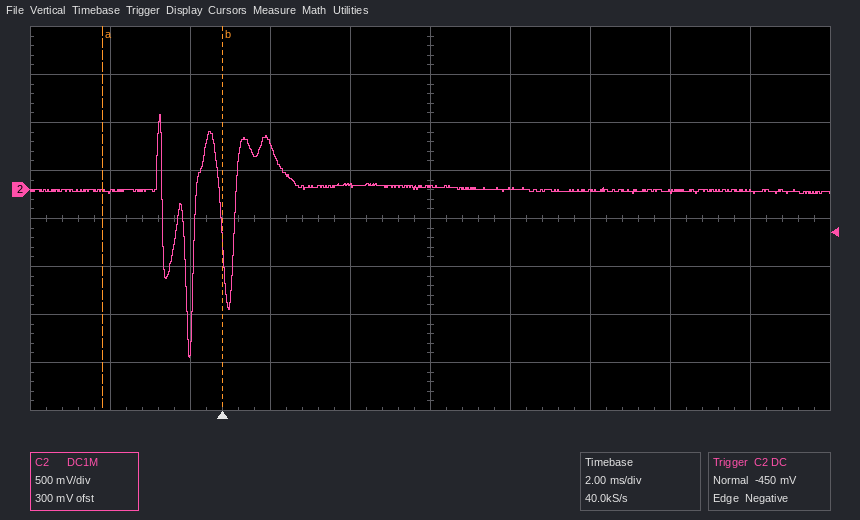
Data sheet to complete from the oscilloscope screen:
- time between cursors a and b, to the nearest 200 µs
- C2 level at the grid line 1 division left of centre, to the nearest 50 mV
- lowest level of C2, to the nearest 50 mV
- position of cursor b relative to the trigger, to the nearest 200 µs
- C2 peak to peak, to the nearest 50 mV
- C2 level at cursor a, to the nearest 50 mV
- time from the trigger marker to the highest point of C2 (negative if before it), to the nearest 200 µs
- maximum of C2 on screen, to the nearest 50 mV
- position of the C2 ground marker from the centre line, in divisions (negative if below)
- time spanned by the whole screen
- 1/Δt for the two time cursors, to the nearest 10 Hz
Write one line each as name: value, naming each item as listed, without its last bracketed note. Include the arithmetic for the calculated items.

time between cursors a and b, to the nearest 200 µs: 3.0 ms
C2 level at the grid line 1 division left of centre, to the nearest 50 mV: 50 mV
lowest level of C2, to the nearest 50 mV: -1.75 V
position of cursor b relative to the trigger, to the nearest 200 µs: 0.0 ms
C2 peak to peak, to the nearest 50 mV: 800 mV − (-1.75 V) = 2.55 V
C2 level at cursor a, to the nearest 50 mV: 0 mV
time from the trigger marker to the highest point of C2 (negative if before it), to the nearest 200 µs: -1.6 ms
maximum of C2 on screen, to the nearest 50 mV: 800 mV
position of the C2 ground marker from the centre line, in divisions: +0.6 div
time spanned by the whole screen: 20 ms
1/Δt for the two time cursors, to the nearest 10 Hz: 1 / 3.0 ms ≈ 330 Hz
